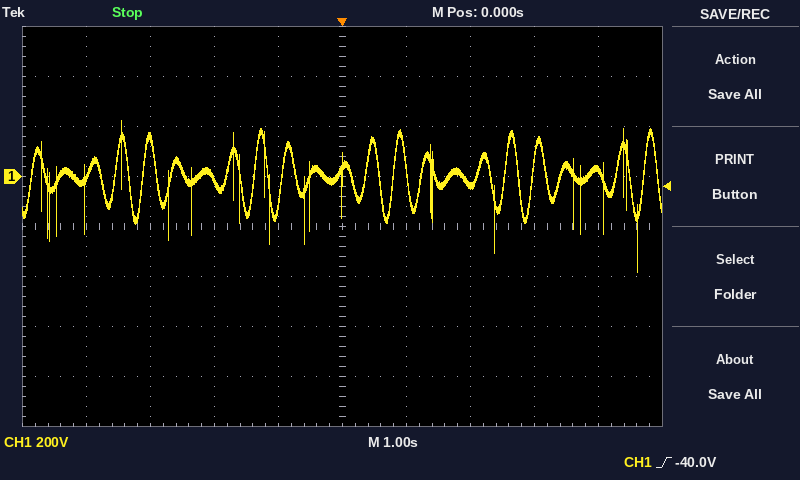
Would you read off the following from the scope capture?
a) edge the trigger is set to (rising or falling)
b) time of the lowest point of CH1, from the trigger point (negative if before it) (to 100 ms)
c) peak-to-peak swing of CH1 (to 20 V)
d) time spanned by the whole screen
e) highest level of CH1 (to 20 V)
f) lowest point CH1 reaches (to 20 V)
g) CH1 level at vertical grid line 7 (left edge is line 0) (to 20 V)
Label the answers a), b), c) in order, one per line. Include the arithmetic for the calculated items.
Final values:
a) rising
b) +4.6 s
c) 220 V − (-380 V) = 600 V
d) 10 s
e) 220 V
f) -380 V
g) -40 V
